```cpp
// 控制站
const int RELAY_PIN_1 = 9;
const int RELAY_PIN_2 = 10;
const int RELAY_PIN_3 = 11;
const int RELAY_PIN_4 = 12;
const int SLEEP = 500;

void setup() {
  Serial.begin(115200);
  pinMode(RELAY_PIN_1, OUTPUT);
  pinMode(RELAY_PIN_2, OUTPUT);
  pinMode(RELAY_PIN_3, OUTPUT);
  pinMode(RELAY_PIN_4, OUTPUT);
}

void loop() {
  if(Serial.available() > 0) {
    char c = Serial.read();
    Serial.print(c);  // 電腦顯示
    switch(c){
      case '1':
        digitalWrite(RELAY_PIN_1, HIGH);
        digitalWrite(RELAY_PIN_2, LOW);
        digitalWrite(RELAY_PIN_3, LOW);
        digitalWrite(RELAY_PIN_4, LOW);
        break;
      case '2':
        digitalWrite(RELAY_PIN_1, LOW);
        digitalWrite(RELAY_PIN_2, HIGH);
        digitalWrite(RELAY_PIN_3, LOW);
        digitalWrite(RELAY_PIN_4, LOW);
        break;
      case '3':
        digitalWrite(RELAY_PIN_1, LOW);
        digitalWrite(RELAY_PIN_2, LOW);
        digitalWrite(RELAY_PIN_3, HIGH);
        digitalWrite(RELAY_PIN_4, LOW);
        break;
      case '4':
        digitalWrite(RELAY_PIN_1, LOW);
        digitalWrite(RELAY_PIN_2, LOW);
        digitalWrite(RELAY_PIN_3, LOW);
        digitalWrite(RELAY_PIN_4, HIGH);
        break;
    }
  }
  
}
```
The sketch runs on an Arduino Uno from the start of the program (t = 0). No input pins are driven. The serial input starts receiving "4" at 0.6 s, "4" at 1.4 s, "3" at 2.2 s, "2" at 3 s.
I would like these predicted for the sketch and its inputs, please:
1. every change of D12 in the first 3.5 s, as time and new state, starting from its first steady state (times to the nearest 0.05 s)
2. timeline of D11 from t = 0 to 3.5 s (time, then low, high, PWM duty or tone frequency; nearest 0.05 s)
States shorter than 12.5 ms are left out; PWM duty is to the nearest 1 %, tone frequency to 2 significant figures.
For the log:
0 s low; 0.6 s high; 2.2 s low
0 s low; 2.2 s high; 3 s low
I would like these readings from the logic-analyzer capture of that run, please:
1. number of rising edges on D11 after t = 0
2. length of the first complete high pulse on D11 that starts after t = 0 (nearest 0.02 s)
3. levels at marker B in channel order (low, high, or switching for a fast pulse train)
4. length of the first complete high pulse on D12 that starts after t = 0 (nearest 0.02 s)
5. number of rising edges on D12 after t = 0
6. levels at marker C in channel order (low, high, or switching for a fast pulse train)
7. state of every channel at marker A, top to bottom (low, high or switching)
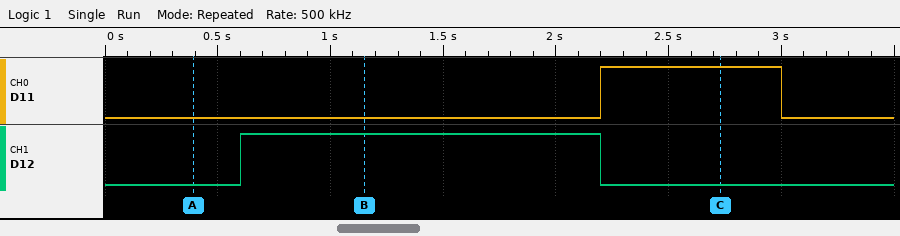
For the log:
1
0.80 s
D11 low, D12 high
1.60 s
1
D11 high, D12 low
D11 low, D12 low
